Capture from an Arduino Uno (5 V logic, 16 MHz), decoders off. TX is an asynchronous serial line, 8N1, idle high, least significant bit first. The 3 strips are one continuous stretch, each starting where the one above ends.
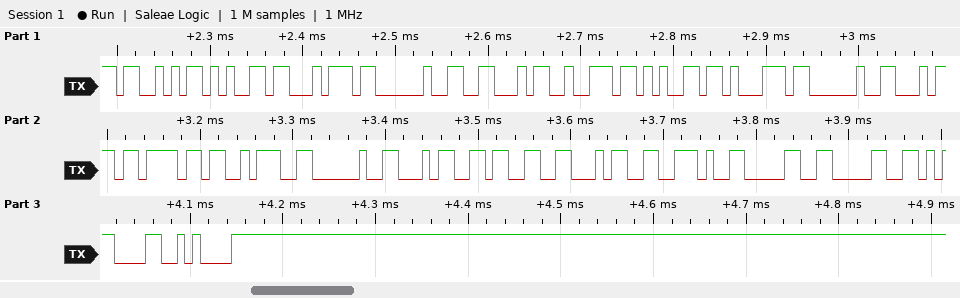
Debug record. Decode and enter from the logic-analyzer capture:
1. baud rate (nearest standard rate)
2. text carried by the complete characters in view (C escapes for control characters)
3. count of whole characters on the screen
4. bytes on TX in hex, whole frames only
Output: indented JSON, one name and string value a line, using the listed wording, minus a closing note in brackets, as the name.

{
  "baud rate": "115200 baud",
  "text carried by the complete characters in view": "\"Set Freq to: 434.00\\r\\n\"",
  "count of whole characters on the screen": "21",
  "bytes on TX in hex, whole frames only": "0x53 0x65 0x74 0x20 0x46 0x72 0x65 0x71 0x20 0x74 0x6F 0x3A 0x20 0x34 0x33 0x34 0x2E 0x30 0x30 0x0D 0x0A"
}
